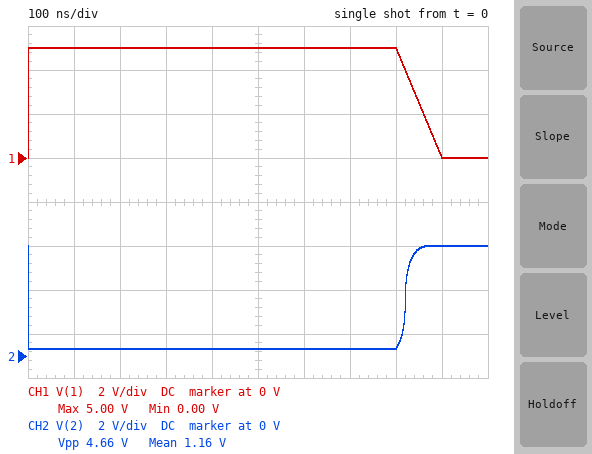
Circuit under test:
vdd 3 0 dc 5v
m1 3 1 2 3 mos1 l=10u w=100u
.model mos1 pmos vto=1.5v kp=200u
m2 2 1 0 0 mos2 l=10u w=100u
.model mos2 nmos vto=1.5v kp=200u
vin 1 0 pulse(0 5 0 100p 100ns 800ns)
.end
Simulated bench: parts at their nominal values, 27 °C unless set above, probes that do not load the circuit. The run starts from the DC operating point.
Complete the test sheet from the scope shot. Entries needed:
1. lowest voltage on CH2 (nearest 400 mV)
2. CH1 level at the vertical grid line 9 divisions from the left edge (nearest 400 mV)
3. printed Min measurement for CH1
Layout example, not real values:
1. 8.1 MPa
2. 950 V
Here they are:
1. 400 mV
2. 0 V
3. 0.00 V
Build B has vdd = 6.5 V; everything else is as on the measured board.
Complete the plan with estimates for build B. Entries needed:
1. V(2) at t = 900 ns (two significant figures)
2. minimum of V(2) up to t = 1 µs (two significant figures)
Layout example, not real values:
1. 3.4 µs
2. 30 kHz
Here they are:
1. 6.5 V
2. 1.7 V
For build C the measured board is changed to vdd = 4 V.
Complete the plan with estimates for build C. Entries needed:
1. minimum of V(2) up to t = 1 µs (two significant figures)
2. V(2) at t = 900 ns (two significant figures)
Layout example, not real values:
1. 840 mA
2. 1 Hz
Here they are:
1. 36 mV
2. 4.0 V
